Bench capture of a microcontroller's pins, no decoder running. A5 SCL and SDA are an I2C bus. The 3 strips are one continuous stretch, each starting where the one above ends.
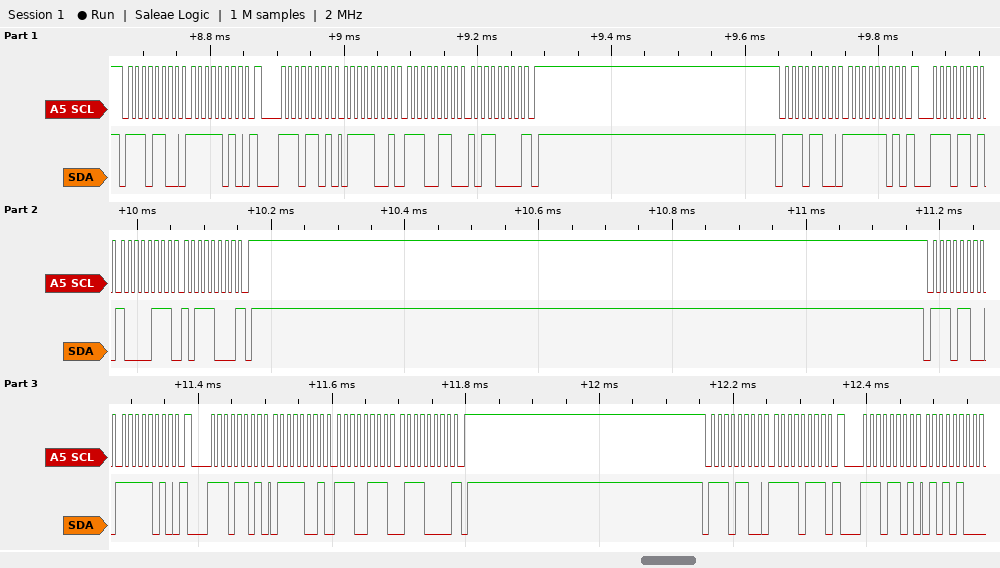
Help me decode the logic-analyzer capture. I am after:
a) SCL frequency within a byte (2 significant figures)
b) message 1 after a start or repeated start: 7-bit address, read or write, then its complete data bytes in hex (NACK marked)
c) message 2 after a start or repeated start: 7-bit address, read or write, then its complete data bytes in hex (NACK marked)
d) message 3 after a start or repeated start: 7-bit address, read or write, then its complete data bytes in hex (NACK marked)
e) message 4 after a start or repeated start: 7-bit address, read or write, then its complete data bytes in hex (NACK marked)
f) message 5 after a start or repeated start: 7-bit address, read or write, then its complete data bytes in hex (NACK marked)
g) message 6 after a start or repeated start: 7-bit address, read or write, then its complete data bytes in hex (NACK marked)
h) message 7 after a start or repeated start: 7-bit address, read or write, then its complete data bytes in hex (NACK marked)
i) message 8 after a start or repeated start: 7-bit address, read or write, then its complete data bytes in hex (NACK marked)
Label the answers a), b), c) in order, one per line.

a) 100 kHz
b) 0x76 write: FA
c) 0x76 read: 79 E6 B0 NACK
d) 0x76 write: FD
e) 0x76 read: 87 B8 NACK
f) 0x76 write: FA
g) 0x76 read: 79 E7 70 NACK
h) 0x76 write: F7
i) 0x76 read: 54
